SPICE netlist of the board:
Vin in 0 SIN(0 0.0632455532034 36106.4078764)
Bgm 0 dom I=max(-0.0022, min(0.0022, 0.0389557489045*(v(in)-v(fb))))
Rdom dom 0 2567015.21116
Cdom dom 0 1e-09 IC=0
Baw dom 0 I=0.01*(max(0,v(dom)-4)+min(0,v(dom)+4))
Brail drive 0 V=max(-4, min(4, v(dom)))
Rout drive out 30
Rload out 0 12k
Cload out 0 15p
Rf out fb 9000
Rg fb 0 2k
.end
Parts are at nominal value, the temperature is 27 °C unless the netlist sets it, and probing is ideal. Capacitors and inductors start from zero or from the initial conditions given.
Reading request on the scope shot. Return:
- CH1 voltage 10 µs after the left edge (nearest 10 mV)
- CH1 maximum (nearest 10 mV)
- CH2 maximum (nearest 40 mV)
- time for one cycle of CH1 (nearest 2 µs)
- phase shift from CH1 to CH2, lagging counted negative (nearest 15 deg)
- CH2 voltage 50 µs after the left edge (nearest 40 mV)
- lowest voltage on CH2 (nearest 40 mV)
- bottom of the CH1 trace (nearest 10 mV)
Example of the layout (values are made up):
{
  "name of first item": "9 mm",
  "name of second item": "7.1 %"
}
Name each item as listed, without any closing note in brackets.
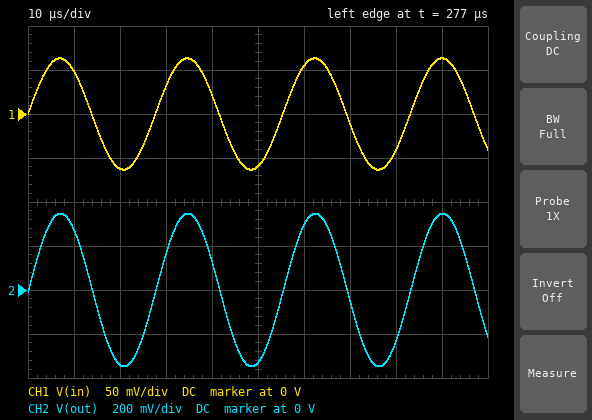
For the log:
{
  "CH1 voltage 10 µs after the left edge": "50 mV",
  "CH1 maximum": "60 mV",
  "CH2 maximum": "360 mV",
  "time for one cycle of CH1": "28 µs",
  "phase shift from CH1 to CH2, lagging counted negative": "0 deg",
  "CH2 voltage 50 µs after the left edge": "-320 mV",
  "lowest voltage on CH2": "-360 mV",
  "bottom of the CH1 trace": "-60 mV"
}
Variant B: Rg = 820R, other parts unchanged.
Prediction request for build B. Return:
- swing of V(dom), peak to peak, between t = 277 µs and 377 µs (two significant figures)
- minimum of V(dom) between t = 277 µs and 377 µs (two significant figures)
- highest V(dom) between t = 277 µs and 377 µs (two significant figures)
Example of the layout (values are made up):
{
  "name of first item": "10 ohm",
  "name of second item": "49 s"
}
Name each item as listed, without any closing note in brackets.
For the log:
{
  "swing of V(dom), peak to peak, between t = 277 µs and 377 µs": "1.5 V",
  "minimum of V(dom) between t = 277 µs and 377 µs": "-760 mV",
  "highest V(dom) between t = 277 µs and 377 µs": "760 mV"
}
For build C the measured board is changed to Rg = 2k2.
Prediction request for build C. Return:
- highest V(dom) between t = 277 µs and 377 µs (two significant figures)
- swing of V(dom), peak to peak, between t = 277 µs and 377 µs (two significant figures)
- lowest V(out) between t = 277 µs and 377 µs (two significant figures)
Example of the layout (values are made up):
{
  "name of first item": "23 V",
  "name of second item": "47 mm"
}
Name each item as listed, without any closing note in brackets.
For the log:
{
  "highest V(dom) between t = 277 µs and 377 µs": "320 mV",
  "swing of V(dom), peak to peak, between t = 277 µs and 377 µs": "650 mV",
  "lowest V(out) between t = 277 µs and 377 µs": "-320 mV"
}
